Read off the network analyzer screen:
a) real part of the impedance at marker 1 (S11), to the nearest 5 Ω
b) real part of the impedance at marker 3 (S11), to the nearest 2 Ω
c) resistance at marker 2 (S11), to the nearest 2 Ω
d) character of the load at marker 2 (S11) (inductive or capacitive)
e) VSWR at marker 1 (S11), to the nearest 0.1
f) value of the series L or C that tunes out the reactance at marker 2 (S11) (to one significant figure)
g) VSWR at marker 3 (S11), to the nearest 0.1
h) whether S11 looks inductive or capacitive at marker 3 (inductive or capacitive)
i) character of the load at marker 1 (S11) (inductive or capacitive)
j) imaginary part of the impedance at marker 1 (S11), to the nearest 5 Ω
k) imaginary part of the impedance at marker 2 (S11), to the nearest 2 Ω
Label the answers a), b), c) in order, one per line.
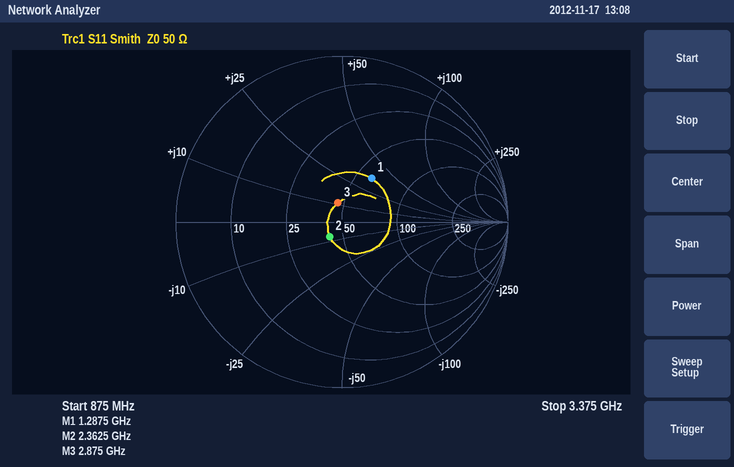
a) 60 Ω
b) 46 Ω
c) 42 Ω
d) capacitive
e) 1.9
f) 500 pH
g) 1.3
h) inductive
i) inductive
j) +35 Ω
k) -8 Ω
